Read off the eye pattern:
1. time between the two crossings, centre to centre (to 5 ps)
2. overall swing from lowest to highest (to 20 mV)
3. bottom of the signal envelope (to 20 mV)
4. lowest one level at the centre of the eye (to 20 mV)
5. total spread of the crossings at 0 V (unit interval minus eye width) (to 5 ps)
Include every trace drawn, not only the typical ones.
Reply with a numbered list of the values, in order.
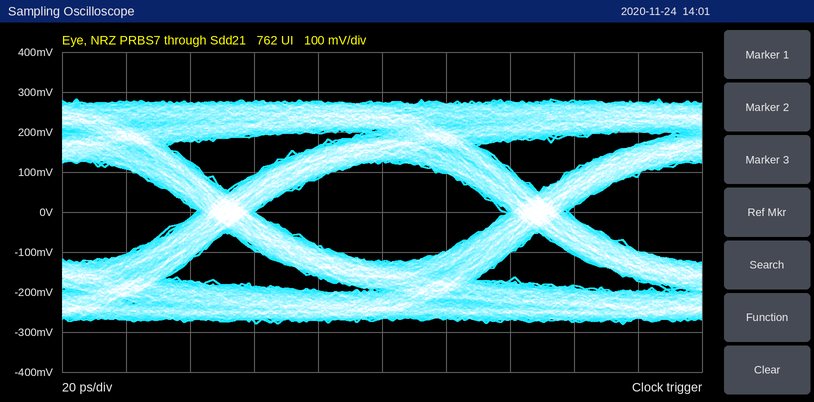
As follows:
1. 95 ps
2. 560 mV
3. -280 mV
4. 120 mV
5. 20 ps
